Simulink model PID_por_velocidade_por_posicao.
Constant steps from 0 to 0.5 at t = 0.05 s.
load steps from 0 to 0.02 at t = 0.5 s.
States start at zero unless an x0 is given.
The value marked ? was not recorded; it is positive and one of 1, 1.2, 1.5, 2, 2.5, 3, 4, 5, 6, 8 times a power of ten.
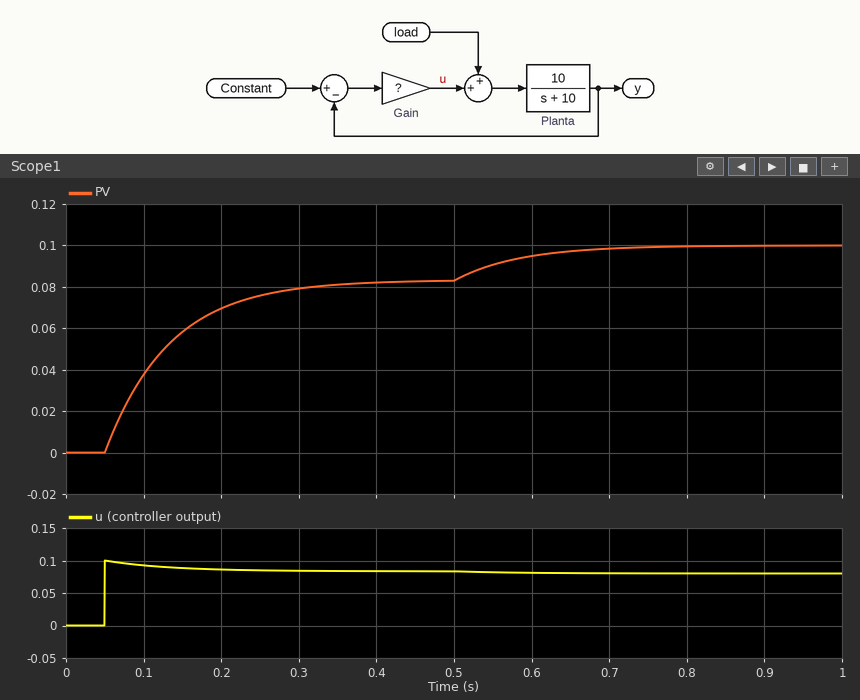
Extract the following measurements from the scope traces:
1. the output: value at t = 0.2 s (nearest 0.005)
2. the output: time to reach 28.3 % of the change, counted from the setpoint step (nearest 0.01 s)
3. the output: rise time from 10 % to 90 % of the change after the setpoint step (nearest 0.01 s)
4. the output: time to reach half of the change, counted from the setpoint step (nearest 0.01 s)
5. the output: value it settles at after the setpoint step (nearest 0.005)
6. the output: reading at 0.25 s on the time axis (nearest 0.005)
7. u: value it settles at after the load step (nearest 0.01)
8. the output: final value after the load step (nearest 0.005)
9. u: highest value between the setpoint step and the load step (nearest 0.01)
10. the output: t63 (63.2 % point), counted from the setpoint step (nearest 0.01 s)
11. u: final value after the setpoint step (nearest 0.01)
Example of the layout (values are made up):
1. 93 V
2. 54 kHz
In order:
1. 0.070
2. 0.03 s
3. 0.18 s
4. 0.06 s
5. 0.085
6. 0.075
7. 0.08
8. 0.100
9. 0.10
10. 0.08 s
11. 0.08
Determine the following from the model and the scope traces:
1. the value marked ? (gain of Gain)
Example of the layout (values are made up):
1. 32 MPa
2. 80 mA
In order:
1. 0.2
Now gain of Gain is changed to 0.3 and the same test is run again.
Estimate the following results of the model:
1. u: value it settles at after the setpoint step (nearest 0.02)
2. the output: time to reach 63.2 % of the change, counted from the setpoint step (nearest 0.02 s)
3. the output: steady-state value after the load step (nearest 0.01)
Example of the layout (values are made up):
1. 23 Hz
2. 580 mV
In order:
1. 0.12
2. 0.08 s
3. 0.13
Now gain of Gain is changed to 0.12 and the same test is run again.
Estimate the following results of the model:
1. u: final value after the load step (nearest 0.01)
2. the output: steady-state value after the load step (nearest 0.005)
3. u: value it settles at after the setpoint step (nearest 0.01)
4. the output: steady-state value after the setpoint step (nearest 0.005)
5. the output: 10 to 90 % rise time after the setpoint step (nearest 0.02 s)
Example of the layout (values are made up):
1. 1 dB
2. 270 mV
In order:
1. 0.05
2. 0.070
3. 0.05
4. 0.055
5. 0.20 s
